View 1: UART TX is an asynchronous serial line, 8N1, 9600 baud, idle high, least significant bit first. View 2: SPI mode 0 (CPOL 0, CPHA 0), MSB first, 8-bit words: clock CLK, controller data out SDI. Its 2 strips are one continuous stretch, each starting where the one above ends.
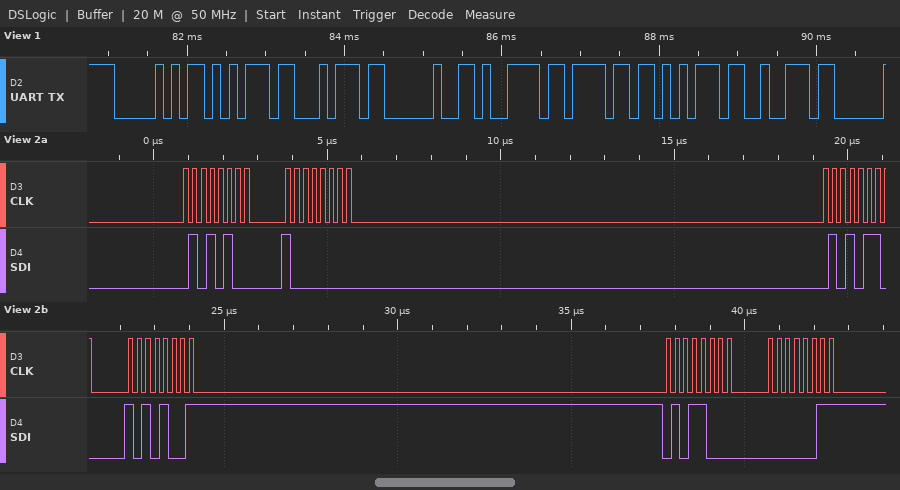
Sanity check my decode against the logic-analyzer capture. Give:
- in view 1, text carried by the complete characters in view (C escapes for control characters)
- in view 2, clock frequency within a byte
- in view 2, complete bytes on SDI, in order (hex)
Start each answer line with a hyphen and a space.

- "Put your"
- 4 MHz
- 0x54 0x80 0x56 0xA9 0x58 0x03
